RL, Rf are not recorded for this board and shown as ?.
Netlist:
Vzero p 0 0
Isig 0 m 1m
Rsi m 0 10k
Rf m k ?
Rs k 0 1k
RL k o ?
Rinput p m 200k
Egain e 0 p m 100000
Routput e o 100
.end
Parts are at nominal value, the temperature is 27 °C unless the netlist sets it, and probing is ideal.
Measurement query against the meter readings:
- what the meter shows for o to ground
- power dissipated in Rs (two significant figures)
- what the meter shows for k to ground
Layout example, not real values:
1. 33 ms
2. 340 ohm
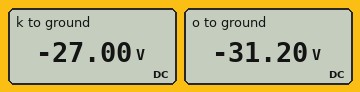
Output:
1. -31.20 V
2. 730 mW
3. -27.00 V
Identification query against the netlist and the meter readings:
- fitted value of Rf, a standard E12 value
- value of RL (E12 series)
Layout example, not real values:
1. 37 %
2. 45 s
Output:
1. 27 kΩ
2. 150 Ω
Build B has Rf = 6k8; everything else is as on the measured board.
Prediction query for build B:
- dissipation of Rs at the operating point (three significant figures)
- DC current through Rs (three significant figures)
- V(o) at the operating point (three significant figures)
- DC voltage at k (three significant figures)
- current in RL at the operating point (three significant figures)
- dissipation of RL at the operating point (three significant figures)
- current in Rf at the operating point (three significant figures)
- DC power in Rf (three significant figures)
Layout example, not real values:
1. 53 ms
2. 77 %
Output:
1. 46.2 mW
2. 6.80 mA
3. -7.97 V
4. -6.80 V
5. 7.80 mA
6. 9.13 mW
7. 1.00 mA
8. 6.80 mW
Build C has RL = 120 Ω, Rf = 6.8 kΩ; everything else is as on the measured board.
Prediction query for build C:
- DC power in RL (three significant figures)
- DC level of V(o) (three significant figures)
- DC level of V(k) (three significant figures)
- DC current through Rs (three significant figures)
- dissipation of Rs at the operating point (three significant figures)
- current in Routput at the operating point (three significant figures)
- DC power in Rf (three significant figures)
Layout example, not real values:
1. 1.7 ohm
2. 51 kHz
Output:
1. 7.30 mW
2. -7.74 V
3. -6.80 V
4. 6.80 mA
5. 46.2 mW
6. 7.80 mA
7. 6.80 mW
